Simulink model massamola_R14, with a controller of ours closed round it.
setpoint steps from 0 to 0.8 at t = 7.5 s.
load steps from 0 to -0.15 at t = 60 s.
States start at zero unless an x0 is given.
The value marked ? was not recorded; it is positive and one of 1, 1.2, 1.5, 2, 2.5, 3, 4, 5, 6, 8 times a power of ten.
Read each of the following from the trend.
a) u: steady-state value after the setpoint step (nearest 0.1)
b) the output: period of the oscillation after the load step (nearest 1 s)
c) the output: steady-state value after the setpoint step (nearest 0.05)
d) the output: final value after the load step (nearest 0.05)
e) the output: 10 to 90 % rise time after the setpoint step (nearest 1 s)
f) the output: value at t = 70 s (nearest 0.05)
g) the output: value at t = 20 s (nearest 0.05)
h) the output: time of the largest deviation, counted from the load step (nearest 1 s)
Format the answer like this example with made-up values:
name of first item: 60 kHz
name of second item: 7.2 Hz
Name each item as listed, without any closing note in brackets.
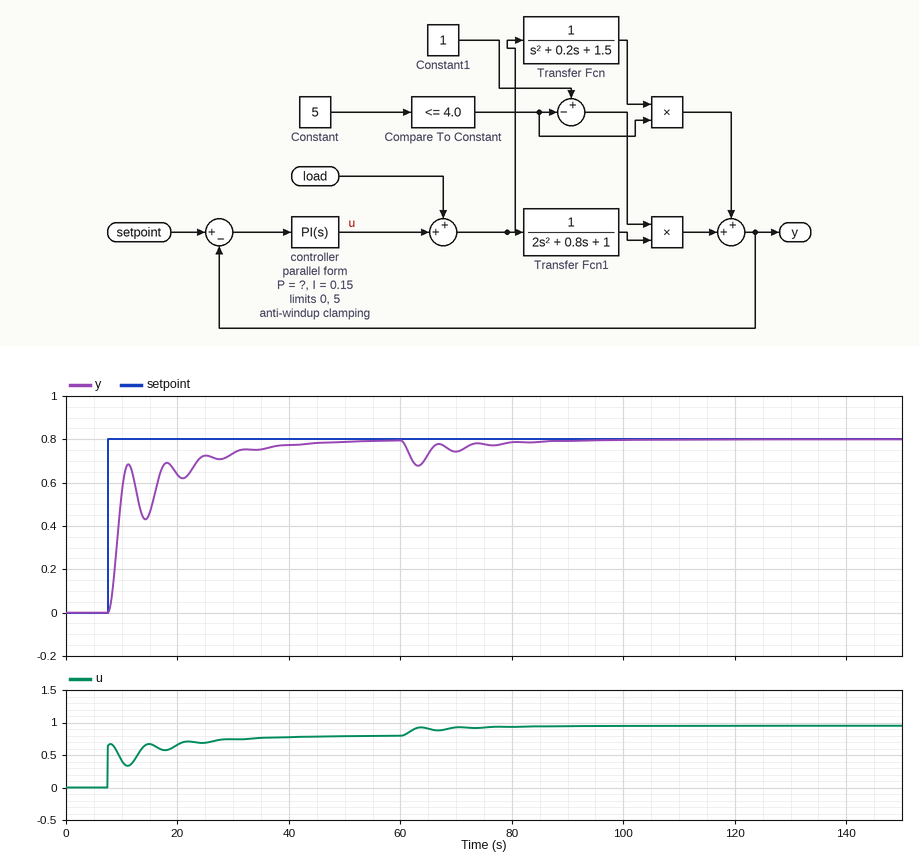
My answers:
u: steady-state value after the setpoint step: 0.8
the output: period of the oscillation after the load step: 7 s
the output: steady-state value after the setpoint step: 0.80
the output: final value after the load step: 0.80
the output: 10 to 90 % rise time after the setpoint step: 16 s
the output: value at t = 70 s: 0.75
the output: value at t = 20 s: 0.65
the output: time of the largest deviation, counted from the load step: 3 s
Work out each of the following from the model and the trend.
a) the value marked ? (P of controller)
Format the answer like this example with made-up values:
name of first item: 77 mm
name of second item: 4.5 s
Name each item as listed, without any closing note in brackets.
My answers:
the value marked ?: 0.8
